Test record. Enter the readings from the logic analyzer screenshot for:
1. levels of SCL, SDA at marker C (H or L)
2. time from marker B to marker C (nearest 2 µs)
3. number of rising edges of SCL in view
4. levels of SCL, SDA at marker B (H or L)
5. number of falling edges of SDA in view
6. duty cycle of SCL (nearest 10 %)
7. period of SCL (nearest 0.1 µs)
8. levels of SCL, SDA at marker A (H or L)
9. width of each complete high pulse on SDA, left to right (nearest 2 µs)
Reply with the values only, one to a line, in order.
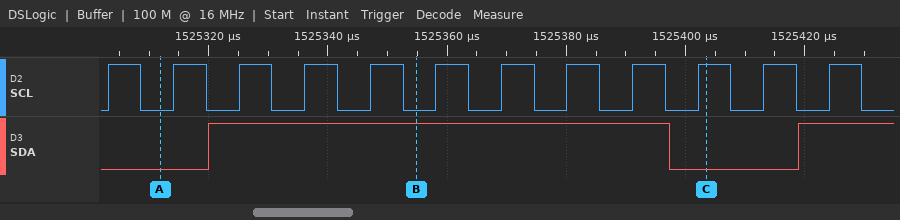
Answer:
SCL=H, SDA=L
48 µs
12
SCL=L, SDA=H
1
50 %
11 µs
SCL=L, SDA=L
78 µs
